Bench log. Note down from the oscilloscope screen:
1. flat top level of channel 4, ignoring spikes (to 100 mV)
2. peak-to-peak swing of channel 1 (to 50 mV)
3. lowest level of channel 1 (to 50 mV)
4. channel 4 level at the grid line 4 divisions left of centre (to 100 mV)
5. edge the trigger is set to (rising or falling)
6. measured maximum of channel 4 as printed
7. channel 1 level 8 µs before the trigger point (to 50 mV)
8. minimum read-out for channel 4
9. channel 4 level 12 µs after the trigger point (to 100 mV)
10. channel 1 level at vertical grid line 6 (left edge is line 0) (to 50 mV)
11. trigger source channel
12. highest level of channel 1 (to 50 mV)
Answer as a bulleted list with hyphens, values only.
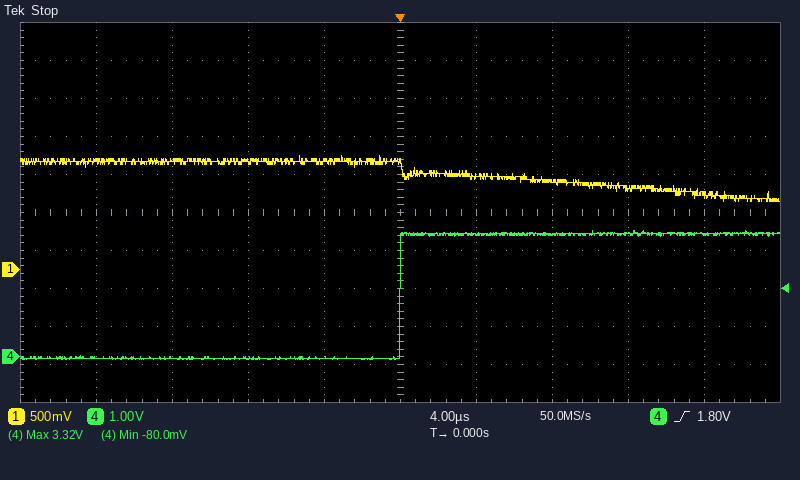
- 3.2 V
- 600 mV
- 900 mV
- 0.0 V
- rising
- 3.32 V
- 1.40 V
- -80.0 mV
- 3.2 V
- 1.20 V
- channel 4
- 1.50 V
